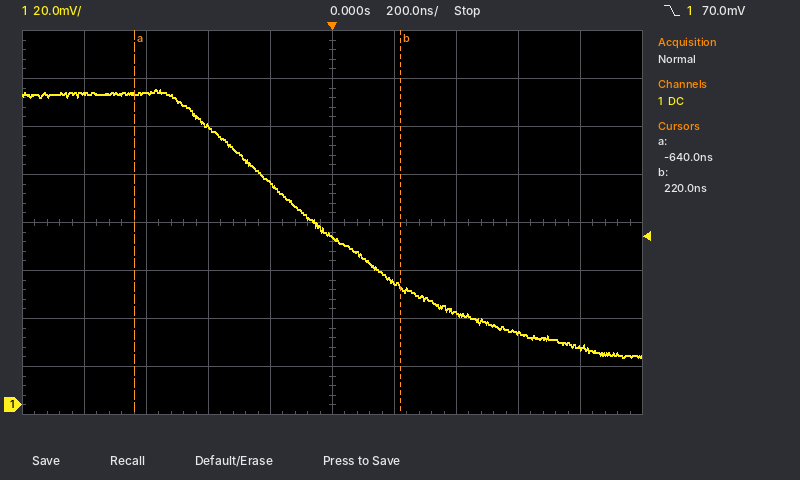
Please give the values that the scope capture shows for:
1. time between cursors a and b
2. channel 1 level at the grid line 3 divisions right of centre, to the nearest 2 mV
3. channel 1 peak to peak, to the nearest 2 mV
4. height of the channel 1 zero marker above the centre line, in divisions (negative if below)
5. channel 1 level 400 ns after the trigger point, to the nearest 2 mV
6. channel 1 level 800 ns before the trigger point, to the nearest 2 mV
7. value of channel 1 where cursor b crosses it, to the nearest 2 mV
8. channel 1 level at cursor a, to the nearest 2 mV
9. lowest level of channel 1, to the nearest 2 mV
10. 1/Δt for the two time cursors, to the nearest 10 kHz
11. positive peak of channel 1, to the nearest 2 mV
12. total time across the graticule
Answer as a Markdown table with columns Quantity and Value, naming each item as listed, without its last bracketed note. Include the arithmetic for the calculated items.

| Quantity | Value |
|---|---|
| time between cursors a and b | 220 ns − (-640 ns) = 860 ns |
| channel 1 level at the grid line 3 divisions right of centre, to the nearest 2 mV | 30 mV |
| channel 1 peak to peak, to the nearest 2 mV | 132 mV − (20 mV) = 112 mV |
| height of the channel 1 zero marker above the centre line, in divisions | -3.8 div |
| channel 1 level 400 ns after the trigger point, to the nearest 2 mV | 38 mV |
| channel 1 level 800 ns before the trigger point, to the nearest 2 mV | 130 mV |
| value of channel 1 where cursor b crosses it, to the nearest 2 mV | 50 mV |
| channel 1 level at cursor a, to the nearest 2 mV | 130 mV |
| lowest level of channel 1, to the nearest 2 mV | 20 mV |
| 1/Δt for the two time cursors, to the nearest 10 kHz | 1 / 860 ns ≈ 1.16 MHz |
| positive peak of channel 1, to the nearest 2 mV | 132 mV |
| total time across the graticule | 2 µs |
